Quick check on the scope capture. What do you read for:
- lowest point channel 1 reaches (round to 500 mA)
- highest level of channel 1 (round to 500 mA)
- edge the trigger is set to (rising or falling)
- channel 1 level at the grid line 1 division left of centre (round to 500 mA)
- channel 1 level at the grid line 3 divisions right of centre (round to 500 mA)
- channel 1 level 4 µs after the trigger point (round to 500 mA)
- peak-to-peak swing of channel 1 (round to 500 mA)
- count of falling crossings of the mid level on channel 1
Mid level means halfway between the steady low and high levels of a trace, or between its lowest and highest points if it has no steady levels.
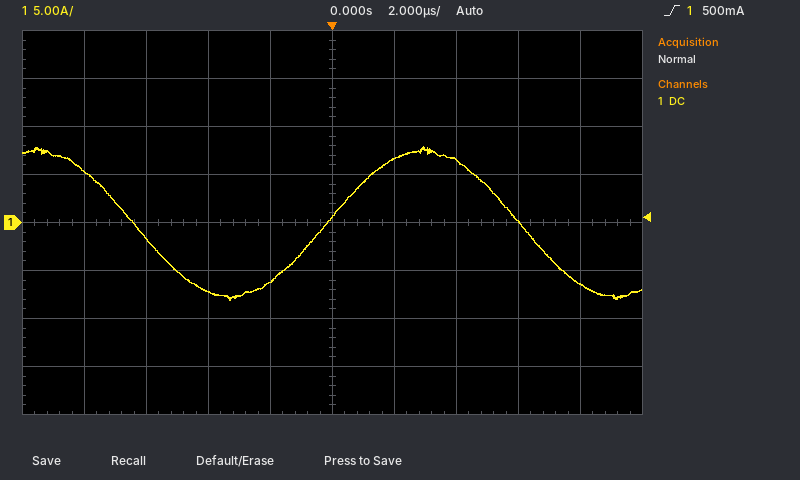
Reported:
-8.0 A
8.0 A
rising
-6.0 A
0.0 A
6.5 A
16.0 A
2
